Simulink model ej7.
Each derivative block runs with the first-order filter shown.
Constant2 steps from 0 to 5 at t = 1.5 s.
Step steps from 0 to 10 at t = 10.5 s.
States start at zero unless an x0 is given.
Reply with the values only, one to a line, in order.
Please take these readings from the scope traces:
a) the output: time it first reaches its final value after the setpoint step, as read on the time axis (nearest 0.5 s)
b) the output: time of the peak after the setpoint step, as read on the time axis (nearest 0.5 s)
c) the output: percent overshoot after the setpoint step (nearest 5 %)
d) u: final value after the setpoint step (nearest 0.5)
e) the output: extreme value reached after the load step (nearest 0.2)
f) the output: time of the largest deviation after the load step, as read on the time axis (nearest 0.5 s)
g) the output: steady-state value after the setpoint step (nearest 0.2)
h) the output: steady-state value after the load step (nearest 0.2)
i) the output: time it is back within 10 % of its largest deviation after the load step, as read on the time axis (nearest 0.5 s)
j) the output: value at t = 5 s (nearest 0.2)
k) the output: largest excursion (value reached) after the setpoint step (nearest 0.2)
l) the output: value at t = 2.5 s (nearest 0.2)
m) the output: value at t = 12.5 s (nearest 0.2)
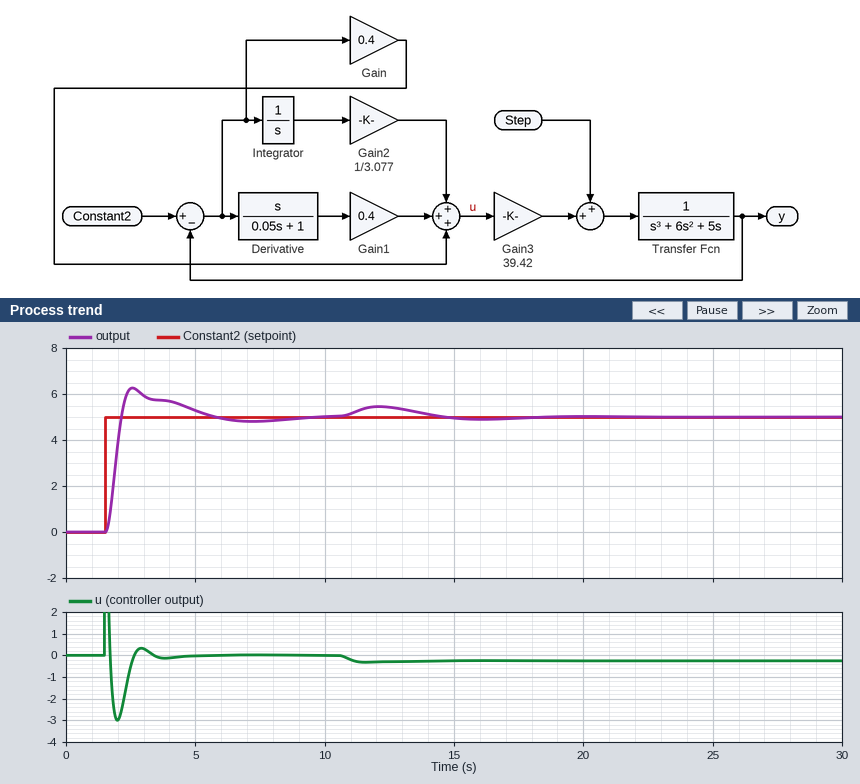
2.0 s
2.5 s
25 %
0.0
5.4
12.0 s
5.0
5.0
17.5 s
5.2
6.2
6.2
5.4
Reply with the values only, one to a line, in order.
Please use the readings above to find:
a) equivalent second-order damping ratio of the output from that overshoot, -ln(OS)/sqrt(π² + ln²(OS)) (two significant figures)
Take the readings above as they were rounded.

0.40
